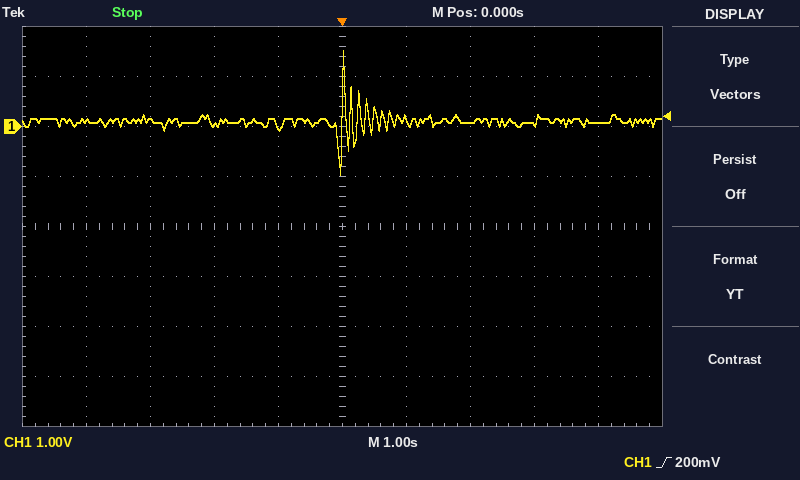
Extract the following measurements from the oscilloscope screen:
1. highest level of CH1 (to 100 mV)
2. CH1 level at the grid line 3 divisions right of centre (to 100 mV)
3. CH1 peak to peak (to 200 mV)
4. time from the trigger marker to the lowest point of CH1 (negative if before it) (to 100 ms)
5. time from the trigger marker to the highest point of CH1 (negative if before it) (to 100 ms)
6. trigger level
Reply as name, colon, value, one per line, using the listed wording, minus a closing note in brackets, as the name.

highest level of CH1: 1.5 V
CH1 level at the grid line 3 divisions right of centre: 100 mV
CH1 peak to peak: 2.4 V
time from the trigger marker to the lowest point of CH1 (negative if before it): 0.0 s
time from the trigger marker to the highest point of CH1 (negative if before it): 0.0 s
trigger level: 200 mV
